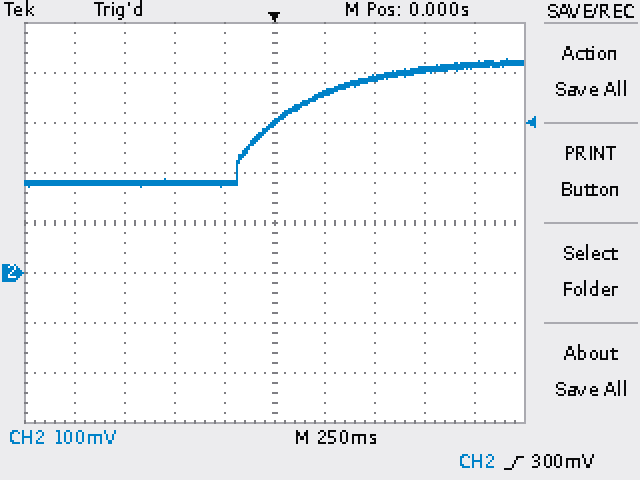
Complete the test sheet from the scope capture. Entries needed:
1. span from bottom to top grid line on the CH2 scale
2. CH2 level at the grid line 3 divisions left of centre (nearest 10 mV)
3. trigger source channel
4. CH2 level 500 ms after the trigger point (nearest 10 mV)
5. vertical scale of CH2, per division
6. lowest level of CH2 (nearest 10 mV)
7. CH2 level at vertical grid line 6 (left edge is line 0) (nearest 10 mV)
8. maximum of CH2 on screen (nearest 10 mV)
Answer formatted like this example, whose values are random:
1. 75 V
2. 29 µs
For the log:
1. 800 mV
2. 180 mV
3. CH2
4. 390 mV
5. 100 mV
6. 170 mV
7. 360 mV
8. 430 mV
